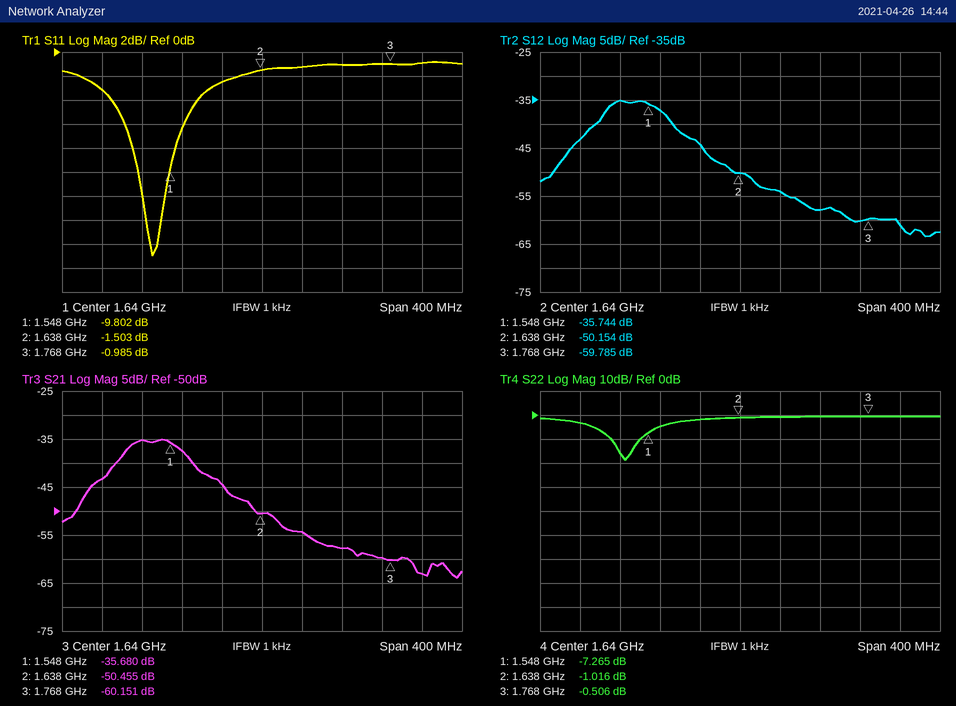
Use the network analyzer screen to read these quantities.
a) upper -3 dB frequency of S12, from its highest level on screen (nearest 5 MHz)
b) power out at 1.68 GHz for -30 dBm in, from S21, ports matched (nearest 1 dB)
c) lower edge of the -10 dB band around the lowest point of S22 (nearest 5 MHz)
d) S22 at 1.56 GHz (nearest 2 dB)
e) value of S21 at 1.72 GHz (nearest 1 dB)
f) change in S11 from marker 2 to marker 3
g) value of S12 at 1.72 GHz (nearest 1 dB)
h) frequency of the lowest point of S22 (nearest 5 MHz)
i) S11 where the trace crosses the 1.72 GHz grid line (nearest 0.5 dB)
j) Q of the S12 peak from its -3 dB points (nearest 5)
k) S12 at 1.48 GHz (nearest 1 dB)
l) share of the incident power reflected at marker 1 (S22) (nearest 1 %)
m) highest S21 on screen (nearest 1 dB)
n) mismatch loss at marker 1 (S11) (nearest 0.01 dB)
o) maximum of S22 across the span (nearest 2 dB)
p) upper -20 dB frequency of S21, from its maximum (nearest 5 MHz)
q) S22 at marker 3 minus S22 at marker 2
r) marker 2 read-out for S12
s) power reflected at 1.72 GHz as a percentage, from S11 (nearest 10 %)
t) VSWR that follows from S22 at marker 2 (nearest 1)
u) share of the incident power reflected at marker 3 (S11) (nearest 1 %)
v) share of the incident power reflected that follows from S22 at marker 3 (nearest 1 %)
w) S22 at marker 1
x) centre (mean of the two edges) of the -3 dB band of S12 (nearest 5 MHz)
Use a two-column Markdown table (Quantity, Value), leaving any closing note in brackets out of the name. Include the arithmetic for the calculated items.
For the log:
| Quantity | Value |
|---|---|
| upper -3 dB frequency of S12, from its highest level on screen | 1.565 GHz |
| power out at 1.68 GHz for -30 dBm in, from S21, ports matched | -30 dBm + (-54 dB) = -84 dBm |
| lower edge of the -10 dB band around the lowest point of S22 | 1.510 GHz |
| S22 at 1.56 GHz | -4 dB |
| value of S21 at 1.72 GHz | -58 dB |
| change in S11 from marker 2 to marker 3 | -0.985 − (-1.503) = 0.518 dB |
| value of S12 at 1.72 GHz | -58 dB |
| frequency of the lowest point of S22 | 1.525 GHz |
| S11 where the trace crosses the 1.72 GHz grid line | -1.0 dB |
| Q of the S12 peak from its -3 dB points | 1.535 GHz / 60 MHz ≈ 25.6, so 25 to the nearest 5 |
| S12 at 1.48 GHz | -43 dB |
| share of the incident power reflected at marker 1 (S22) | 10^(-7.265/10) ≈ 19 % |
| highest S21 on screen | -35 dB |
| mismatch loss at marker 1 (S11) | −10 log10(1 − 10^(-9.802/10)) ≈ 0.48 dB |
| maximum of S22 across the span | 0 dB |
| upper -20 dB frequency of S21, from its maximum | 1.685 GHz |
| S22 at marker 3 minus S22 at marker 2 | -0.506 − (-1.016) = 0.510 dB |
| marker 2 read-out for S12 | -50.154 dB |
| power reflected at 1.72 GHz as a percentage, from S11 | 10^(-1/10) ≈ 79.4 %, so 80 % to the nearest 10 % |
| VSWR that follows from S22 at marker 2 | (1 + 0.8896)/(1 − 0.8896) ≈ 17 |
| share of the incident power reflected at marker 3 (S11) | 10^(-0.985/10) ≈ 80 % |
| share of the incident power reflected that follows from S22 at marker 3 | 10^(-0.506/10) ≈ 89 % |
| S22 at marker 1 | -7.265 dB |
| centre (mean of the two edges) of the -3 dB band of S12 | 1.535 GHz |
